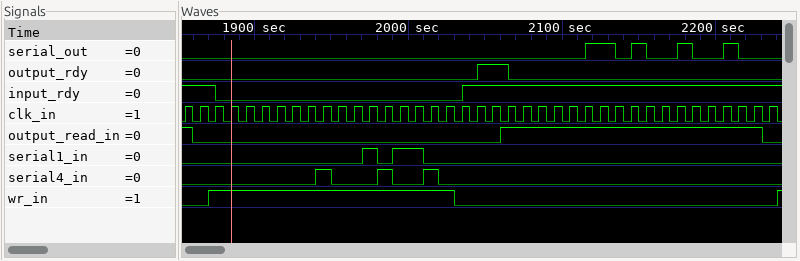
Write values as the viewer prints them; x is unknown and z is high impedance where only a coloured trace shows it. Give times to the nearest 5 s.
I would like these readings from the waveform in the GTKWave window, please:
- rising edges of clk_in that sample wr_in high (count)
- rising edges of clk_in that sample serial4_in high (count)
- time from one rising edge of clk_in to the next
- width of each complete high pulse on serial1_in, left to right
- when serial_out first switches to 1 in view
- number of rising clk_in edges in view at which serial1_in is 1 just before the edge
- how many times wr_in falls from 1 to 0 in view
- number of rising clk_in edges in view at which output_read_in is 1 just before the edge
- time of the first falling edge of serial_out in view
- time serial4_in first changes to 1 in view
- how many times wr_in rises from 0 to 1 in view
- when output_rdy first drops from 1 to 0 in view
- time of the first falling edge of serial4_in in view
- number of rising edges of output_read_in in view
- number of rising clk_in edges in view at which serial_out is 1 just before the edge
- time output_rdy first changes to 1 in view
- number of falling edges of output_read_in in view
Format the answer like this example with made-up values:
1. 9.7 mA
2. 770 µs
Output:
1. 16
2. 3
3. 10 s
4. 10 s, 20 s
5. 2115 s
6. 3
7. 1
8. 18
9. 2135 s
10. 1940 s
11. 2
12. 2065 s
13. 1950 s
14. 1
15. 5
16. 2045 s
17. 2
